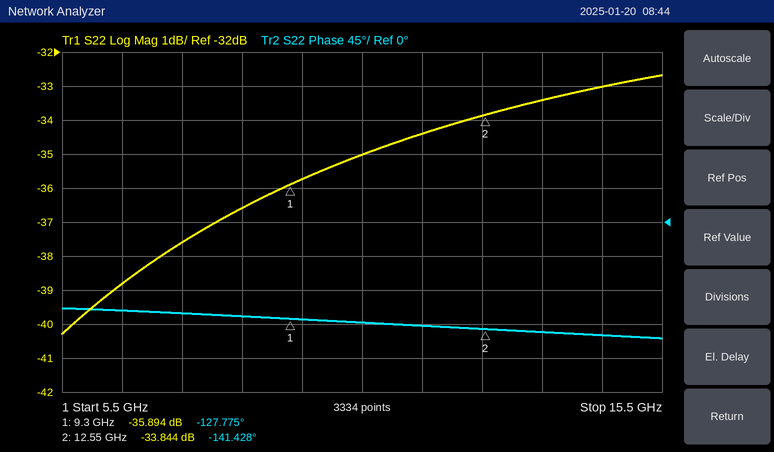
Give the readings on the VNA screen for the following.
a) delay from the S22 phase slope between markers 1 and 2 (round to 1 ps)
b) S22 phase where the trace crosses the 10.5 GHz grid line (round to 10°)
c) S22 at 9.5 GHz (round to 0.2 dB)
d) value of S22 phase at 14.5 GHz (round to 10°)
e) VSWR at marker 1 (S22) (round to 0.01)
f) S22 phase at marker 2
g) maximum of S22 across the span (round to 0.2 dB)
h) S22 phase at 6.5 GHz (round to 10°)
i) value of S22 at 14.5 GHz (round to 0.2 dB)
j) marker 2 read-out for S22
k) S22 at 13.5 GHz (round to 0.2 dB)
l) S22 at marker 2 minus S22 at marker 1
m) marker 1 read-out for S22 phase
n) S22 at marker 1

12 ps
-130°
-35.8 dB
-150°
1.03
-141.428°
-32.6 dB
-120°
-33.0 dB
-33.844 dB
-33.4 dB
2.050 dB
-127.775°
-35.894 dB
